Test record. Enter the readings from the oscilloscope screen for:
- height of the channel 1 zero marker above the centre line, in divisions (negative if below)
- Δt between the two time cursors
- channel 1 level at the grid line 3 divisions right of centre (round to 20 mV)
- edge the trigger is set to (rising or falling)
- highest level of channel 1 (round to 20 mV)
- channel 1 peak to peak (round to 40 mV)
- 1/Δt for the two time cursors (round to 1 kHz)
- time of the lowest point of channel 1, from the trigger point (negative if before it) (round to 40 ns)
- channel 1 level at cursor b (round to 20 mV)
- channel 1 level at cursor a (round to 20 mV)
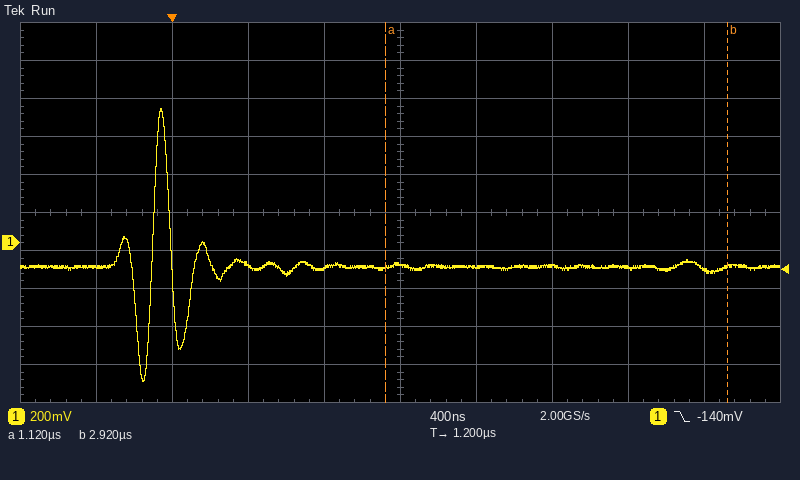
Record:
-0.8 div
1.80 µs
-140 mV
falling
700 mV
1.44 V
556 kHz
-160 ns
-120 mV
-140 mV
